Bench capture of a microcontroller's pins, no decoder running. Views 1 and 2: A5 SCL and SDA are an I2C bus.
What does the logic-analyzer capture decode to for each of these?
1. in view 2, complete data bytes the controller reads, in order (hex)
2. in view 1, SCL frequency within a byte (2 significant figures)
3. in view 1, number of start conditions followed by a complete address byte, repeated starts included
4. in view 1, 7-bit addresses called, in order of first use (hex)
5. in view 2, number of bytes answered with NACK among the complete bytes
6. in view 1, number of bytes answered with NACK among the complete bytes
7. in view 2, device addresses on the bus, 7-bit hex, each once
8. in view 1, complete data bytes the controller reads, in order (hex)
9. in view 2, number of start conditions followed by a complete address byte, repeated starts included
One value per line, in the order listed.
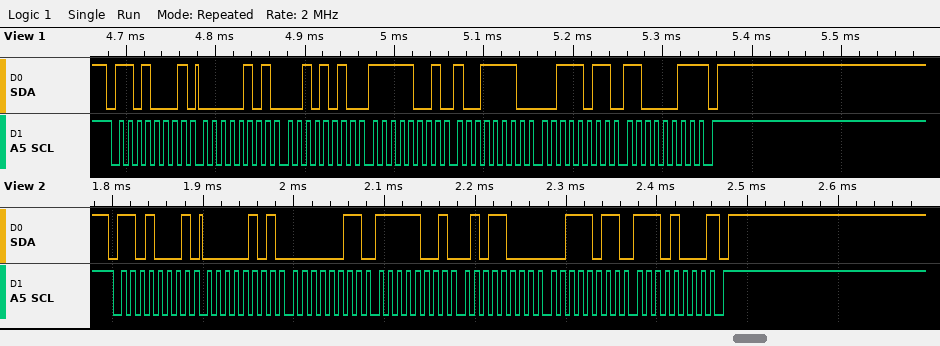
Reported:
05 03 F9 58 3B E8
100 kHz
1
0x68
1
1
0x68
05 2A F9 9E 3B C3
1
